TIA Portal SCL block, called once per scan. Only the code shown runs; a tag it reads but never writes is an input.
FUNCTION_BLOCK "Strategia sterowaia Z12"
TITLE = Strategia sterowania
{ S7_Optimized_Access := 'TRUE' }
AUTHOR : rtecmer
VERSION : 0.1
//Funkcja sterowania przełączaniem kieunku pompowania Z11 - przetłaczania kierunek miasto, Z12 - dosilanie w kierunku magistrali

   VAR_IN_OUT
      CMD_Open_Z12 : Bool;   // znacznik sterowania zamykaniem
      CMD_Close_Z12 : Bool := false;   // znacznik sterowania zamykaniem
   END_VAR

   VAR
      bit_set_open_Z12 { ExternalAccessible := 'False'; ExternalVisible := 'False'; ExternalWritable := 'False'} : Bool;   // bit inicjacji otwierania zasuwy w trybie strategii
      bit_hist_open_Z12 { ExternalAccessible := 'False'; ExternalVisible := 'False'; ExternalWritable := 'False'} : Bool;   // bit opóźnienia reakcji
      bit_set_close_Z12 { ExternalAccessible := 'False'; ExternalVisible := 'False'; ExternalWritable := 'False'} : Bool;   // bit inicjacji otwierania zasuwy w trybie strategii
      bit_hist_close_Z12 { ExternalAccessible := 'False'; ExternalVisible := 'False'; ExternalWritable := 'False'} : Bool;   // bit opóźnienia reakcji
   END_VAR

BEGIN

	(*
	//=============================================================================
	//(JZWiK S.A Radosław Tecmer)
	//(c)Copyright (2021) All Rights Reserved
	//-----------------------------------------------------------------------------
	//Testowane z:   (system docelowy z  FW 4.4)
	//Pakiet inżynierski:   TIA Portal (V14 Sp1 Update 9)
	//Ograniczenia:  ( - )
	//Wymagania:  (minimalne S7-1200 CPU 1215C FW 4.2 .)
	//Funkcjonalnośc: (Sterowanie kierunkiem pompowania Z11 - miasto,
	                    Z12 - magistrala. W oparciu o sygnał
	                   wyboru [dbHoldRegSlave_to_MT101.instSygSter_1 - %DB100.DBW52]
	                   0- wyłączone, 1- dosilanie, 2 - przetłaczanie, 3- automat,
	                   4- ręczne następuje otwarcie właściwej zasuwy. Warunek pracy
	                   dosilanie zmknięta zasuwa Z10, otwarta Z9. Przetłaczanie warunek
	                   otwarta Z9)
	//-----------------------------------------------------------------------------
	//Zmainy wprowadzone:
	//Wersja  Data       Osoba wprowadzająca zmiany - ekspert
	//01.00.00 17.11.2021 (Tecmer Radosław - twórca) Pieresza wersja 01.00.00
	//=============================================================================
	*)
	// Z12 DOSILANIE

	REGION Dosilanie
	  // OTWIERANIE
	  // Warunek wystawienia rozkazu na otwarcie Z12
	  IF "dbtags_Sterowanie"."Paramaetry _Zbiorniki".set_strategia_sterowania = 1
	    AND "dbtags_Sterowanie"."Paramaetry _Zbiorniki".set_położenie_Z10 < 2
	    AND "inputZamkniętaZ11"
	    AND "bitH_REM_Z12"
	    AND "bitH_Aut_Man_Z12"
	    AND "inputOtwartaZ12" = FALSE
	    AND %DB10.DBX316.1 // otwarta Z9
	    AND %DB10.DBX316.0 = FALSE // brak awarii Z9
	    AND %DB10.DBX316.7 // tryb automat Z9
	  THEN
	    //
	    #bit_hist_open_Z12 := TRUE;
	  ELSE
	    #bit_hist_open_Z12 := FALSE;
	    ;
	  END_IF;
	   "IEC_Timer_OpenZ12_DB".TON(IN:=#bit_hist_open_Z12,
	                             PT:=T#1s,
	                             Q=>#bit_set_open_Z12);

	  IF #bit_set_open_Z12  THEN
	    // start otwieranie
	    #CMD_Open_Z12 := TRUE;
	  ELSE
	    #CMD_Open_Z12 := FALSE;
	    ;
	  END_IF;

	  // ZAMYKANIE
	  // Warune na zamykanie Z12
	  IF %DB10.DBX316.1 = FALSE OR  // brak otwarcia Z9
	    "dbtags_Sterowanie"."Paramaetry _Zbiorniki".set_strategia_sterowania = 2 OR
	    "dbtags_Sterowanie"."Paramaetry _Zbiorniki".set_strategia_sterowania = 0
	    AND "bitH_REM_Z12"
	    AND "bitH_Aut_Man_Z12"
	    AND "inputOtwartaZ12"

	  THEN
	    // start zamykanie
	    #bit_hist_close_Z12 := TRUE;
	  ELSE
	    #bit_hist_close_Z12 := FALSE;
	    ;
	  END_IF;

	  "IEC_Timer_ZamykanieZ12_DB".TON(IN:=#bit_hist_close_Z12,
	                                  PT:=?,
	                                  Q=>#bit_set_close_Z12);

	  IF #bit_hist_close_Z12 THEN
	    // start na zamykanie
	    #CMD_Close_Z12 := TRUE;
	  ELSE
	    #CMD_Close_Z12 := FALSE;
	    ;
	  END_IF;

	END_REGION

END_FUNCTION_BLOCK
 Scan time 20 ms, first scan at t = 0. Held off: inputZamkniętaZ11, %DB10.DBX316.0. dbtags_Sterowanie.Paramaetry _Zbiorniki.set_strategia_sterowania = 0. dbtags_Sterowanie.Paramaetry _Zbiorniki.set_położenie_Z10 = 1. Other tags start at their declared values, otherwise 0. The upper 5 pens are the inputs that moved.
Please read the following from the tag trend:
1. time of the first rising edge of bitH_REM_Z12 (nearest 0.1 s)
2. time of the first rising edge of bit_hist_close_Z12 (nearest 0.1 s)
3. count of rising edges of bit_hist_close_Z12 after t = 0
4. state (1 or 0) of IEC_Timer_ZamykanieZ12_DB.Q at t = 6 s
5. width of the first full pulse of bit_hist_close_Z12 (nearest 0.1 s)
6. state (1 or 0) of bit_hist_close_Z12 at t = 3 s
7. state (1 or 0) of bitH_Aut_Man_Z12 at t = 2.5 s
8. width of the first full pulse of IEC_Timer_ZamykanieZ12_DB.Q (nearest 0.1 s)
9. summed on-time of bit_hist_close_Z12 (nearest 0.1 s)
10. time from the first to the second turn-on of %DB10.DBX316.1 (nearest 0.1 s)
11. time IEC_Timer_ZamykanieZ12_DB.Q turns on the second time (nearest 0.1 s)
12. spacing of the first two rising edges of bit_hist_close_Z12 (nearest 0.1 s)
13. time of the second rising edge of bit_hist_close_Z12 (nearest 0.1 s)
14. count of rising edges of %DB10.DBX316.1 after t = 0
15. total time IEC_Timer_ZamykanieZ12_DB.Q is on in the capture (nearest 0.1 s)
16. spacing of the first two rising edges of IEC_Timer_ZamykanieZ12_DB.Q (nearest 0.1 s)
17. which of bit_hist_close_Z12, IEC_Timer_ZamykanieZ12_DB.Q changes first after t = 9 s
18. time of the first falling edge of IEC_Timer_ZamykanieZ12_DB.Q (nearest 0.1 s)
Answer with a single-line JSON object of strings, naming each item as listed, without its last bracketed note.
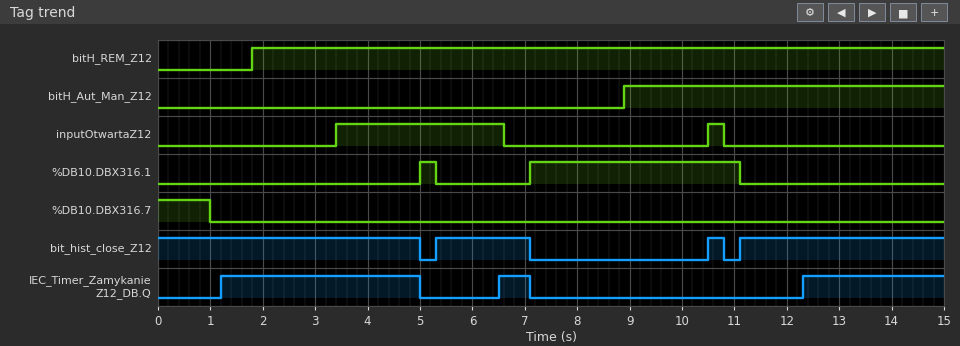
{"time of the first rising edge of bitH_REM_Z12": "1.8 s", "time of the first rising edge of bit_hist_close_Z12": "5.3 s", "count of rising edges of bit_hist_close_Z12 after t = 0": "3", "state (1 or 0) of IEC_Timer_ZamykanieZ12_DB.Q at t = 6 s": "0", "width of the first full pulse of bit_hist_close_Z12": "1.8 s", "state (1 or 0) of bit_hist_close_Z12 at t = 3 s": "1", "state (1 or 0) of bitH_Aut_Man_Z12 at t = 2.5 s": "0", "width of the first full pulse of IEC_Timer_ZamykanieZ12_DB.Q": "3.8 s", "summed on-time of bit_hist_close_Z12": "11.0 s", "time from the first to the second turn-on of %DB10.DBX316.1": "2.1 s", "time IEC_Timer_ZamykanieZ12_DB.Q turns on the second time": "6.5 s", "spacing of the first two rising edges of bit_hist_close_Z12": "5.2 s", "time of the second rising edge of bit_hist_close_Z12": "10.5 s", "count of rising edges of %DB10.DBX316.1 after t = 0": "2", "total time IEC_Timer_ZamykanieZ12_DB.Q is on in the capture": "7.1 s", "spacing of the first two rising edges of IEC_Timer_ZamykanieZ12_DB.Q": "5.3 s", "which of bit_hist_close_Z12, IEC_Timer_ZamykanieZ12_DB.Q changes first after t = 9 s": "bit_hist_close_Z12", "time of the first falling edge of IEC_Timer_ZamykanieZ12_DB.Q": "5.0 s"}
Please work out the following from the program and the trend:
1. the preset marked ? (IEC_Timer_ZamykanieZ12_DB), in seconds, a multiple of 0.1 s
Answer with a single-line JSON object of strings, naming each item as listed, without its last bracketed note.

{"the preset marked ? (IEC_Timer_ZamykanieZ12_DB), in seconds, a multiple of 0.1 s": "1.2 s"}
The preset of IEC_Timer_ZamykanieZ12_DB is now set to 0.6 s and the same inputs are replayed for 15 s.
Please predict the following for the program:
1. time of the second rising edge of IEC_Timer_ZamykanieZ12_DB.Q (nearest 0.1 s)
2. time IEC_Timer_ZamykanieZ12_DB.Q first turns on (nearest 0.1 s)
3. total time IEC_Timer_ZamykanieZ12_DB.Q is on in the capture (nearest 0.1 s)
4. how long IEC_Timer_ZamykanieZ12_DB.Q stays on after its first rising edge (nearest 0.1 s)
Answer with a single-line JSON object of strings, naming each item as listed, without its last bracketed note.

{"time of the second rising edge of IEC_Timer_ZamykanieZ12_DB.Q": "5.9 s", "time IEC_Timer_ZamykanieZ12_DB.Q first turns on": "0.6 s", "total time IEC_Timer_ZamykanieZ12_DB.Q is on in the capture": "8.9 s", "how long IEC_Timer_ZamykanieZ12_DB.Q stays on after its first rising edge": "4.4 s"}
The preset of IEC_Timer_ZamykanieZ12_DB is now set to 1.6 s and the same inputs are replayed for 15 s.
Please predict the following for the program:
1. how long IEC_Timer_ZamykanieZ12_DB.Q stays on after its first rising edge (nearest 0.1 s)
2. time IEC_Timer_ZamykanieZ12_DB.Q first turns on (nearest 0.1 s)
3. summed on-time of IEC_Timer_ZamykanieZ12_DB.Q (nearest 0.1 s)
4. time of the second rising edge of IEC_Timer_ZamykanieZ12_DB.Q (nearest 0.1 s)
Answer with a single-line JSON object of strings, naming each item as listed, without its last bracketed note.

{"how long IEC_Timer_ZamykanieZ12_DB.Q stays on after its first rising edge": "3.4 s", "time IEC_Timer_ZamykanieZ12_DB.Q first turns on": "1.6 s", "summed on-time of IEC_Timer_ZamykanieZ12_DB.Q": "5.9 s", "time of the second rising edge of IEC_Timer_ZamykanieZ12_DB.Q": "6.9 s"}
